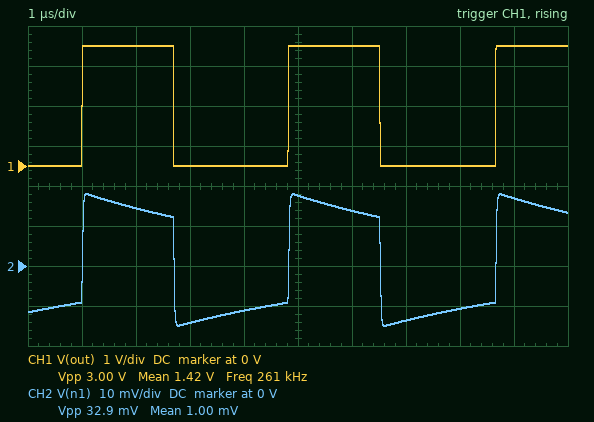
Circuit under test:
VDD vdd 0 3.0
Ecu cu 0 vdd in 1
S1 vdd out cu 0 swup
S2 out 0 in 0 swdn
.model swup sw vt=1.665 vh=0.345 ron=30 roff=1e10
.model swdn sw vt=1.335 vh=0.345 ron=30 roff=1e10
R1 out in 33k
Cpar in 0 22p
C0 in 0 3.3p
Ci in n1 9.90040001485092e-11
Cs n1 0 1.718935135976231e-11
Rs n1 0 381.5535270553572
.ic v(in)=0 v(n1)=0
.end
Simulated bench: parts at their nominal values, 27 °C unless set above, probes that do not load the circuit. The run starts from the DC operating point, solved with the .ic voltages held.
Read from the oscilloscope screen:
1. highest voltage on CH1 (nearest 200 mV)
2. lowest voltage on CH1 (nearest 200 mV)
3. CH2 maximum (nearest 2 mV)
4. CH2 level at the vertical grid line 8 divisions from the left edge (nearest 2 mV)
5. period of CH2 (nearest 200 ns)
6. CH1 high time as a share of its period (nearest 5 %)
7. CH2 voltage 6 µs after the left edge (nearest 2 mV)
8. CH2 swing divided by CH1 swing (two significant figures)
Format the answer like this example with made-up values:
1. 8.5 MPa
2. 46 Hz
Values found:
1. 3.0 V
2. 0 V
3. 18 mV
4. -10 mV
5. 3.8 µs
6. 45 %
7. 14 mV
8. 0.011
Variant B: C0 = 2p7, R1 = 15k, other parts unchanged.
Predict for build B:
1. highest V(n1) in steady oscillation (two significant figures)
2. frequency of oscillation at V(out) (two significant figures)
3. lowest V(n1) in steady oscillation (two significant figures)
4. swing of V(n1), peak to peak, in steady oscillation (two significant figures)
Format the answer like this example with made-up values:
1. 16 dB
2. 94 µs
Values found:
1. 38 mV
2. 590 kHz
3. -32 mV
4. 70 mV
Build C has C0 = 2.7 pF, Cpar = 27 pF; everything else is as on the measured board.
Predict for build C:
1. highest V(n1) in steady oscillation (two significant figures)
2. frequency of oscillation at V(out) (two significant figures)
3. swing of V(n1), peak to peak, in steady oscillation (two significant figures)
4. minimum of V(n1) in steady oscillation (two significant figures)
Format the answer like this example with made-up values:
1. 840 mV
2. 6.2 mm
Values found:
1. 17 mV
2. 250 kHz
3. 32 mV
4. -14 mV
